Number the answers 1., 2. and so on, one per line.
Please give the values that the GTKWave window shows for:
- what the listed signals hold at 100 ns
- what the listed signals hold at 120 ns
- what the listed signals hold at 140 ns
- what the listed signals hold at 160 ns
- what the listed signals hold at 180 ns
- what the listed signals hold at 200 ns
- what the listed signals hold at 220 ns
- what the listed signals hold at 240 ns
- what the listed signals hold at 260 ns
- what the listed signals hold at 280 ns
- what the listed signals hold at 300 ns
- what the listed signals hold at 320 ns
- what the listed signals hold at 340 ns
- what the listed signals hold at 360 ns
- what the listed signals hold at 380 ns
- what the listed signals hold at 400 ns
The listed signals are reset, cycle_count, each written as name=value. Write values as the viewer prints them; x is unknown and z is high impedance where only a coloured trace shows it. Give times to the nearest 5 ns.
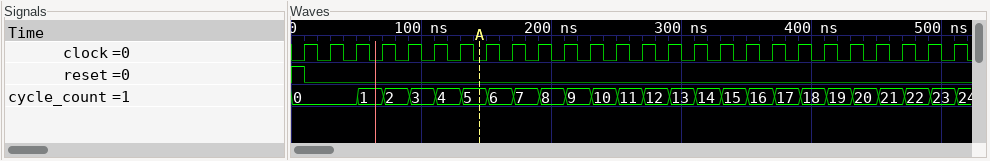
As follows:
1. reset=0, cycle_count=3
2. reset=0, cycle_count=4
3. reset=0, cycle_count=5
4. reset=0, cycle_count=6
5. reset=0, cycle_count=7
6. reset=0, cycle_count=8
7. reset=0, cycle_count=9
8. reset=0, cycle_count=10
9. reset=0, cycle_count=11
10. reset=0, cycle_count=12
11. reset=0, cycle_count=13
12. reset=0, cycle_count=14
13. reset=0, cycle_count=15
14. reset=0, cycle_count=16
15. reset=0, cycle_count=17
16. reset=0, cycle_count=18
